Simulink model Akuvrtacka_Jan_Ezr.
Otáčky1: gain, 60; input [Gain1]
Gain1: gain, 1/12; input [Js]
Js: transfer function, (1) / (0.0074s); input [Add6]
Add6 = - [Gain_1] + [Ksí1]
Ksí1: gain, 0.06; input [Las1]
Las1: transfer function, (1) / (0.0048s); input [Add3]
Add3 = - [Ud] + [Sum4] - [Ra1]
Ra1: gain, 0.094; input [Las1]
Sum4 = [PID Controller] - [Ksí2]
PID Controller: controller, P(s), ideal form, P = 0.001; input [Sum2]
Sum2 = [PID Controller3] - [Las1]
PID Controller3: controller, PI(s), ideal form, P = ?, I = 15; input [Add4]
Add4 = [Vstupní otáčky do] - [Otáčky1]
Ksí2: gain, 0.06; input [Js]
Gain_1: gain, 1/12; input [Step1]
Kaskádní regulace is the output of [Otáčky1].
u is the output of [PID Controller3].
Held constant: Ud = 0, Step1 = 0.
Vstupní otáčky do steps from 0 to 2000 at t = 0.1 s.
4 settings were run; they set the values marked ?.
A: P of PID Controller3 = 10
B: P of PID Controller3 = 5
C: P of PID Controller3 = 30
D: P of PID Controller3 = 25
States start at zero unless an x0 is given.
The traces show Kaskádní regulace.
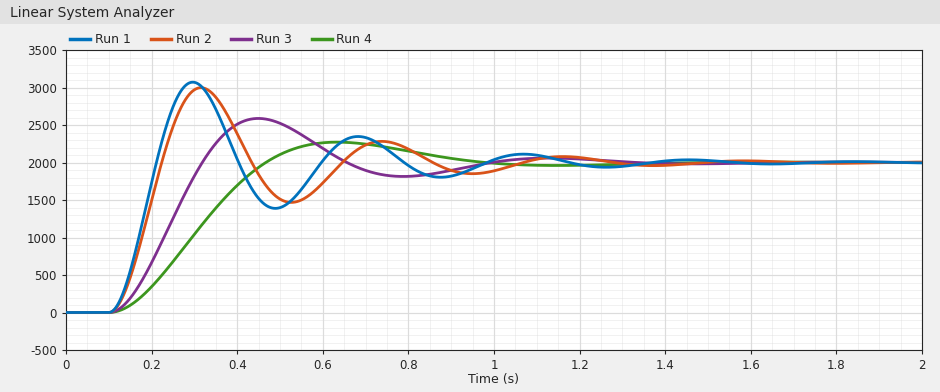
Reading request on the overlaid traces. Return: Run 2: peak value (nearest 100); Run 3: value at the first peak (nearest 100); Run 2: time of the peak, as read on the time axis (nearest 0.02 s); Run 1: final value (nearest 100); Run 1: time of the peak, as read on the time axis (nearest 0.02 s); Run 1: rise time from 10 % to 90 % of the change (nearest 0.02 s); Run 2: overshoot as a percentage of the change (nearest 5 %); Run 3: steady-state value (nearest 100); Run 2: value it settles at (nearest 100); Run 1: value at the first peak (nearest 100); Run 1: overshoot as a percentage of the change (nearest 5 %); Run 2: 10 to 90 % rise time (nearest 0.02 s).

3000
2600
0.32 s
2000
0.30 s
0.08 s
50 %
2000
2000
3100
55 %
0.08 s
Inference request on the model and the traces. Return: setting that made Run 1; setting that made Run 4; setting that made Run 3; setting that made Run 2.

C
B
A
D
